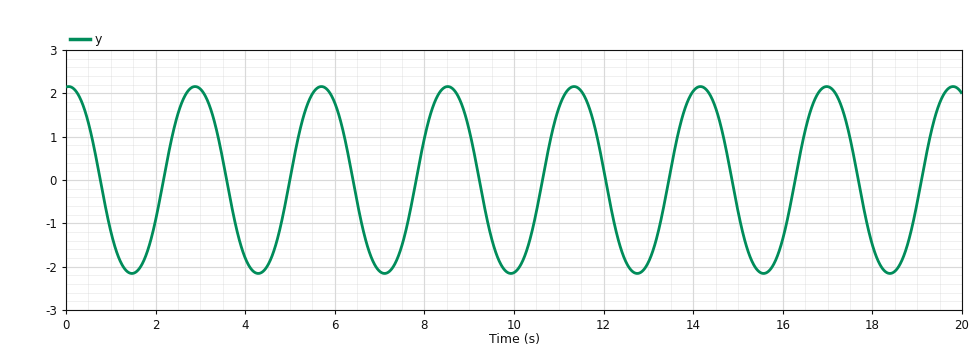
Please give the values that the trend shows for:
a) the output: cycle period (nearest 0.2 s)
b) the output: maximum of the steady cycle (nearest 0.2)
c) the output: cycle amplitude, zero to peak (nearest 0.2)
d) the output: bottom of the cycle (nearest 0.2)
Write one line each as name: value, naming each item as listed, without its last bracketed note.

the output: cycle period: 2.8 s
the output: maximum of the steady cycle: 2.2
the output: cycle amplitude, zero to peak: 2.2
the output: bottom of the cycle: -2.2
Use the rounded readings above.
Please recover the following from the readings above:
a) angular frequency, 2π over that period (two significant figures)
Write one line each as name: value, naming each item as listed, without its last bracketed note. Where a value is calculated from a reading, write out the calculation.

angular frequency, 2π over that period: 2π / 2.8 = 2.2 rad/s
